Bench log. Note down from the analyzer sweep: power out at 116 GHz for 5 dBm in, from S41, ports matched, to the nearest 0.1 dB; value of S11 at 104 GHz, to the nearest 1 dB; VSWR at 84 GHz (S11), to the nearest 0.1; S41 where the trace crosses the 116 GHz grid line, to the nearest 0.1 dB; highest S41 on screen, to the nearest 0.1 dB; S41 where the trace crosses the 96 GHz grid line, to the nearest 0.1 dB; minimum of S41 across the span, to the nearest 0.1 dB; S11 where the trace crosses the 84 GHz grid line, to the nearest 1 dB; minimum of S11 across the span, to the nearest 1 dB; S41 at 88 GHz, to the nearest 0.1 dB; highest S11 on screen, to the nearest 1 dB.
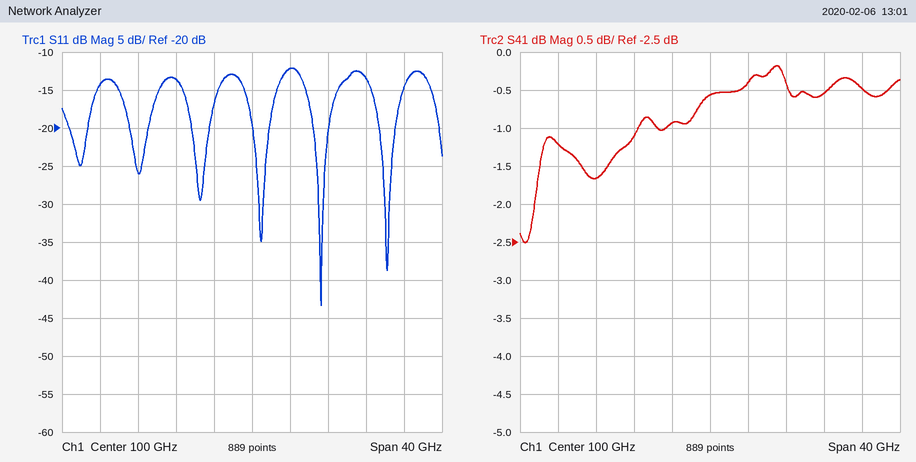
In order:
4.5 dBm
-12 dB
1.5
-0.5 dB
-0.2 dB
-0.9 dB
-2.5 dB
-14 dB
-43 dB
-1.7 dB
-12 dB
